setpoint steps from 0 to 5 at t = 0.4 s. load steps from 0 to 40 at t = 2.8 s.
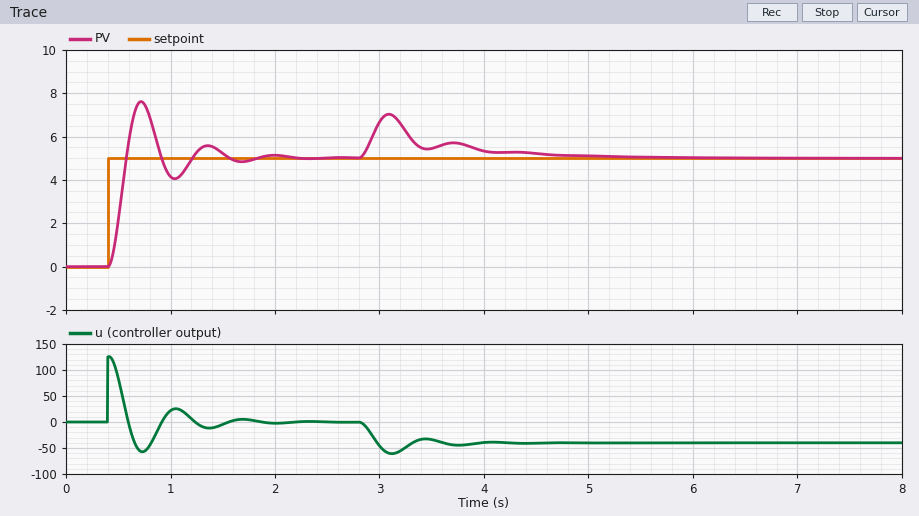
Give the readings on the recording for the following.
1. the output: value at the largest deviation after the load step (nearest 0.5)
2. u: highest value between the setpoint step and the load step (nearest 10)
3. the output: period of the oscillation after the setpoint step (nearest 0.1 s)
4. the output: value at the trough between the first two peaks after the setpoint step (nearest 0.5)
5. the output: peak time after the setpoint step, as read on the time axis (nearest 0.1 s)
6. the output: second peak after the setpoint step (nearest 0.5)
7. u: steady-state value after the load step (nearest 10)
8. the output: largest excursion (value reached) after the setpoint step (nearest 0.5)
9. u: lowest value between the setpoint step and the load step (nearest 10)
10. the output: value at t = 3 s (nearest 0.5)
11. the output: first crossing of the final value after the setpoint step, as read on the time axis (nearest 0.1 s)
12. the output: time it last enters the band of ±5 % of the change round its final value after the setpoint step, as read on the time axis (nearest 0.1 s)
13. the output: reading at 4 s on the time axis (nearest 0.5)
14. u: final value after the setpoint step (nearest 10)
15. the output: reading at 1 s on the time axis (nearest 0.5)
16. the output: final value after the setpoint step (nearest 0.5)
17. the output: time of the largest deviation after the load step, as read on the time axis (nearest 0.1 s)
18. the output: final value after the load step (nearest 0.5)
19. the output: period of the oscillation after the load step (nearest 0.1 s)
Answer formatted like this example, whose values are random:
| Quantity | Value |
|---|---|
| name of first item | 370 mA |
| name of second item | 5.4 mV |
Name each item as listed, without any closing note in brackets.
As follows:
| Quantity | Value |
|---|---|
| the output: value at the largest deviation after the load step | 7.0 |
| u: highest value between the setpoint step and the load step | 130 |
| the output: period of the oscillation after the setpoint step | 0.6 s |
| the output: value at the trough between the first two peaks after the setpoint step | 4.0 |
| the output: peak time after the setpoint step, as read on the time axis | 0.7 s |
| the output: second peak after the setpoint step | 5.5 |
| u: steady-state value after the load step | -40 |
| the output: largest excursion (value reached) after the setpoint step | 7.5 |
| u: lowest value between the setpoint step and the load step | -60 |
| the output: value at t = 3 s | 6.5 |
| the output: first crossing of the final value after the setpoint step, as read on the time axis | 0.6 s |
| the output: time it last enters the band of ±5 % of the change round its final value after the setpoint step, as read on the time axis | 1.5 s |
| the output: reading at 4 s on the time axis | 5.5 |
| u: final value after the setpoint step | 0 |
| the output: reading at 1 s on the time axis | 4.0 |
| the output: final value after the setpoint step | 5.0 |
| the output: time of the largest deviation after the load step, as read on the time axis | 3.1 s |
| the output: final value after the load step | 5.0 |
| the output: period of the oscillation after the load step | 0.6 s |
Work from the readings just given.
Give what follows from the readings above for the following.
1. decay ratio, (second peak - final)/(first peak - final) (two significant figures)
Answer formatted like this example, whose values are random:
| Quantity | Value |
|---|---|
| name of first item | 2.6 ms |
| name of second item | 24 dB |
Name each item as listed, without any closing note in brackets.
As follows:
| Quantity | Value |
|---|---|
| decay ratio, (second peak - final)/(first peak - final) | 0.20 |
